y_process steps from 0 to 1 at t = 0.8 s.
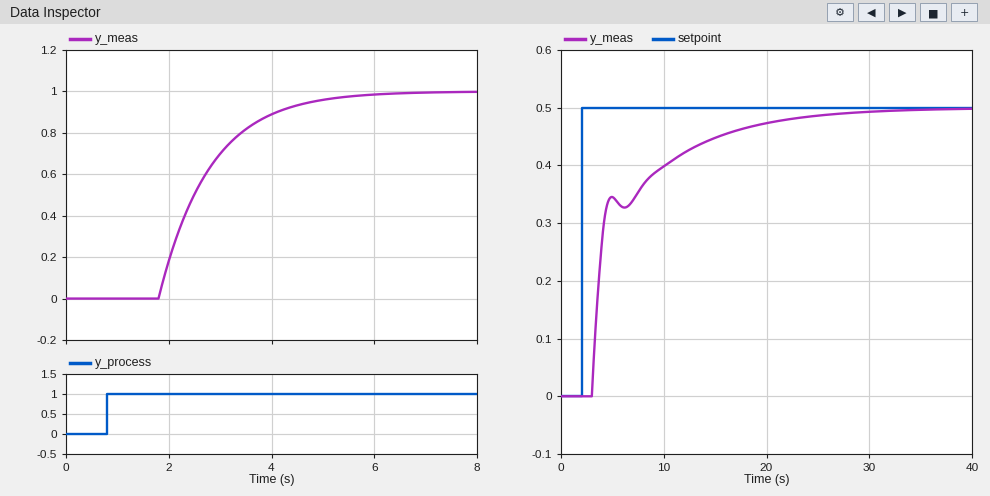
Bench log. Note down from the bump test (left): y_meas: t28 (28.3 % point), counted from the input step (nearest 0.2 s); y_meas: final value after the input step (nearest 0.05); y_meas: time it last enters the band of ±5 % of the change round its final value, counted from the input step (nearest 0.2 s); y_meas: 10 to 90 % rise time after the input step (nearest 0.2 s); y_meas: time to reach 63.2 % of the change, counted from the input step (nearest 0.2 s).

1.4 s
1.00
4.0 s
2.2 s
2.0 s
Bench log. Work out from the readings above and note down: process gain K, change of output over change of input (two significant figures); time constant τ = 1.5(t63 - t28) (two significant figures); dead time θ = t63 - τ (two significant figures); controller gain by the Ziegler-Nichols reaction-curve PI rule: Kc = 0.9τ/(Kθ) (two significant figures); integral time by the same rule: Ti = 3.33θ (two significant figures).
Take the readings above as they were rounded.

1.0
0.90 s
1.1 s
0.74
3.7 s
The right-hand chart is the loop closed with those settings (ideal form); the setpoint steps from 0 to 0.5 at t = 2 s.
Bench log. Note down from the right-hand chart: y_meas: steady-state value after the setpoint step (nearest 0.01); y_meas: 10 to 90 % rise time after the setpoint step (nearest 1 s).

0.50
12 s
